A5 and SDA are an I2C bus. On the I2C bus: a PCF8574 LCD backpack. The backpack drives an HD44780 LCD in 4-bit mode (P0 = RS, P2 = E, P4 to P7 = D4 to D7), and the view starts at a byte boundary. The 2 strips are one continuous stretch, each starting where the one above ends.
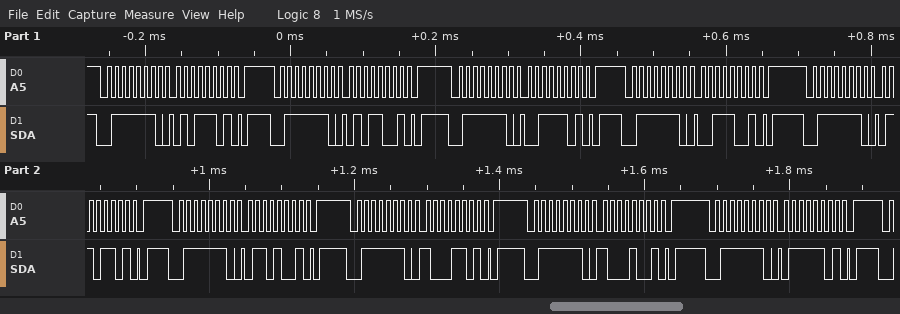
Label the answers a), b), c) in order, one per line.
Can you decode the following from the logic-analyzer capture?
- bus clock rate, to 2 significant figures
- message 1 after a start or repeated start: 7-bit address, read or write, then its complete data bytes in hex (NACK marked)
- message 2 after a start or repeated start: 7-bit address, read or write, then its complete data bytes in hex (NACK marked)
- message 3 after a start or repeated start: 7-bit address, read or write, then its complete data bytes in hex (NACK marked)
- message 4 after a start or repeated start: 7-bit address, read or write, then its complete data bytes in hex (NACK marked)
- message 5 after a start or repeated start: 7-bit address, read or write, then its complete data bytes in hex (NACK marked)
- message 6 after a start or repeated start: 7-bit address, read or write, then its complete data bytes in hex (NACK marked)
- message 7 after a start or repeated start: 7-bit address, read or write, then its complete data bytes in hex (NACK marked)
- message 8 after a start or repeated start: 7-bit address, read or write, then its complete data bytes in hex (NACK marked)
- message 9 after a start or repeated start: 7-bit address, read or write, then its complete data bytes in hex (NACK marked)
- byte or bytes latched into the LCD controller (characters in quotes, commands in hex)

a) 100 kHz
b) 0x3F write: 5D
c) 0x3F write: 59
d) 0x3F write: 3D
e) 0x3F write: 39
f) 0x3F write: 6D
g) 0x3F write: 69
h) 0x3F write: 8D
i) 0x3F write: 89
j) 0x3F write: 7D
k) 'S' 'h'
